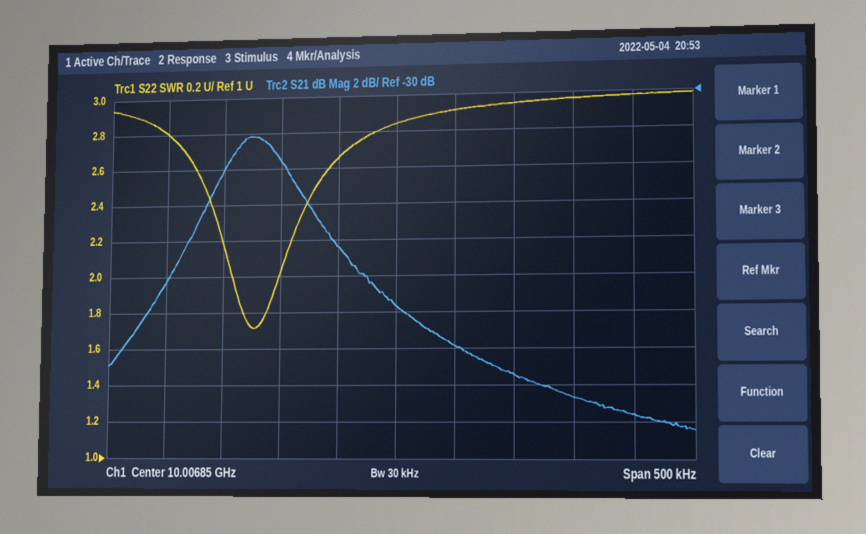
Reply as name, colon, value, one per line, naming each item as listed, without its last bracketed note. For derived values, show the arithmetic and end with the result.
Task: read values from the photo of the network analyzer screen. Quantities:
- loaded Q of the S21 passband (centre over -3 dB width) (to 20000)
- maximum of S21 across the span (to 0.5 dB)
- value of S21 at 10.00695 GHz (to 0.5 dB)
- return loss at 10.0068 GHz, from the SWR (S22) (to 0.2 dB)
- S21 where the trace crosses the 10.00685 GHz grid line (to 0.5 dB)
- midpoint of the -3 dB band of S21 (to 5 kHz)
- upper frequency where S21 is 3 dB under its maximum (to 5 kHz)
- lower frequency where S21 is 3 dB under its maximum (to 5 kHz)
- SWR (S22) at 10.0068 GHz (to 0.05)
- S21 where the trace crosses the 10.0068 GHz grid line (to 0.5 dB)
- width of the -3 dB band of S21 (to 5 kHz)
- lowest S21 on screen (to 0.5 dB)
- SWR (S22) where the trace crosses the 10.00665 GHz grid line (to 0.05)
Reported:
loaded Q of the S21 passband (centre over -3 dB width): 10.0067 GHz / 75 kHz ≈ 133423, so 140000 to the nearest 20000
maximum of S21 across the span: -32.0 dB
value of S21 at 10.00695 GHz: -45.5 dB
return loss at 10.0068 GHz, from the SWR (S22): −20 log10((2.65 − 1)/(2.65 + 1)) ≈ 6.90 dB, so 6.8 dB to the nearest 0.2 dB
S21 where the trace crosses the 10.00685 GHz grid line: -41.5 dB
midpoint of the -3 dB band of S21: 10.006730 GHz
upper frequency where S21 is 3 dB under its maximum: 10.006765 GHz
lower frequency where S21 is 3 dB under its maximum: 10.006690 GHz
SWR (S22) at 10.0068 GHz: 2.65
S21 where the trace crosses the 10.0068 GHz grid line: -38.5 dB
width of the -3 dB band of S21: 10.006765 GHz − 10.006690 GHz = 75 kHz
lowest S21 on screen: -48.5 dB
SWR (S22) where the trace crosses the 10.00665 GHz grid line: 2.80
